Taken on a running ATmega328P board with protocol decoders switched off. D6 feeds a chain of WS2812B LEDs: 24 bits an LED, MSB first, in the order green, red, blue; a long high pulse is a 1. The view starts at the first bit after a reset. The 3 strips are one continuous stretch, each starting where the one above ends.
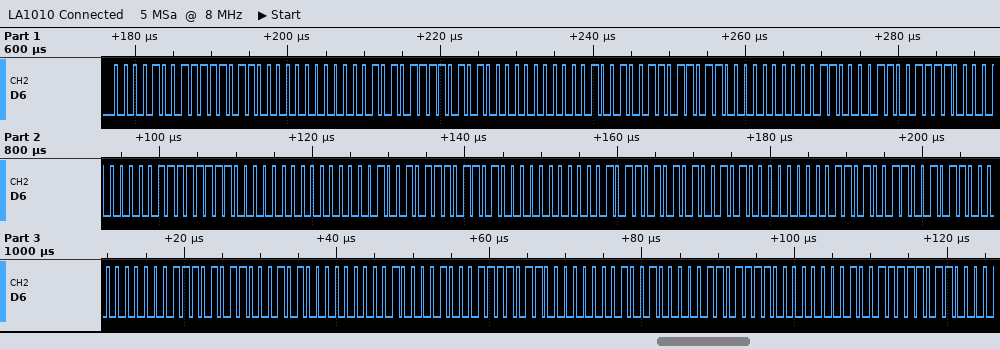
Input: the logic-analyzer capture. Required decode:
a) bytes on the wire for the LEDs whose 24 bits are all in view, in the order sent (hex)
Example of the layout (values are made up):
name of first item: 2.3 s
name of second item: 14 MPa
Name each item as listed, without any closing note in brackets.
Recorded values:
bytes on the wire for the LEDs whose 24 bits are all in view, in the order sent: 09 F6 00 15 EA 00 24 DB 00 30 CF 00 3F C0 00 4B B4 00 5A A5 00 69 96 00 75 8A 00 84 7B 00 90 6F 00
